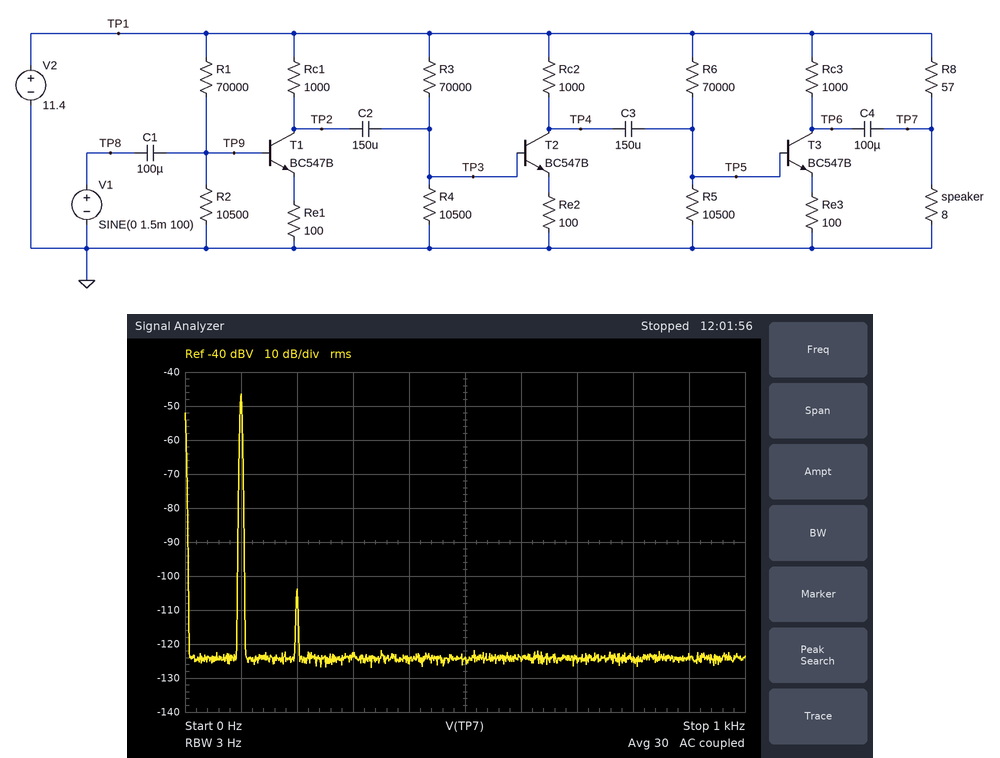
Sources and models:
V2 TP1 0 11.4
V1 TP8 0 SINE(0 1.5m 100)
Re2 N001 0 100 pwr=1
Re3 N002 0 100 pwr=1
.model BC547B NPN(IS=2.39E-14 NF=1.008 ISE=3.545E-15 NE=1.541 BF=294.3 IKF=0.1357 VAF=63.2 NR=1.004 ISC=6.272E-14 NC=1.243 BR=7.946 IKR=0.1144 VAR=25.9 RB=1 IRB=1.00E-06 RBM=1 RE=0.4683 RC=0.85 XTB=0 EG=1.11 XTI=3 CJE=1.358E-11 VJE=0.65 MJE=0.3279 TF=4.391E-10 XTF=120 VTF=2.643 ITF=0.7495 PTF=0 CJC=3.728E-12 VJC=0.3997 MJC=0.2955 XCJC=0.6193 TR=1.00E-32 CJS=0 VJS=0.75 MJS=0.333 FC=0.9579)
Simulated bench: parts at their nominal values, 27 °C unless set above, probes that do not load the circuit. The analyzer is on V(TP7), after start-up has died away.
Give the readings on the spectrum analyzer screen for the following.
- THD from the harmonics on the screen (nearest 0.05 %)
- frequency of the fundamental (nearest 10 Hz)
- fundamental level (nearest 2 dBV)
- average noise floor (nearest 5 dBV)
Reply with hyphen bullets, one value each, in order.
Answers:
- 0.15 %
- 100 Hz
- -46 dBV
- -125 dBV
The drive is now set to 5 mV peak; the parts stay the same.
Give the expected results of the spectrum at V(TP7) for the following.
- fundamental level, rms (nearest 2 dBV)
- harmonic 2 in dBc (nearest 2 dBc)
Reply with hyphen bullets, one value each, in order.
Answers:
- -36 dBV
- -46 dBc
